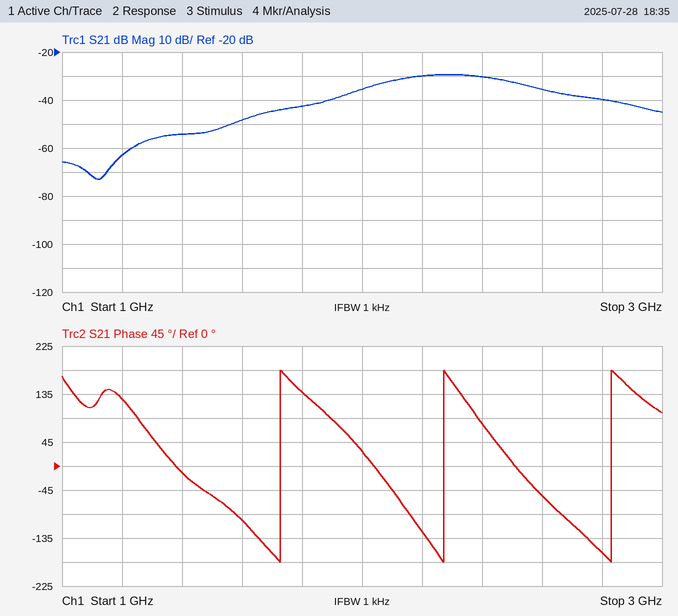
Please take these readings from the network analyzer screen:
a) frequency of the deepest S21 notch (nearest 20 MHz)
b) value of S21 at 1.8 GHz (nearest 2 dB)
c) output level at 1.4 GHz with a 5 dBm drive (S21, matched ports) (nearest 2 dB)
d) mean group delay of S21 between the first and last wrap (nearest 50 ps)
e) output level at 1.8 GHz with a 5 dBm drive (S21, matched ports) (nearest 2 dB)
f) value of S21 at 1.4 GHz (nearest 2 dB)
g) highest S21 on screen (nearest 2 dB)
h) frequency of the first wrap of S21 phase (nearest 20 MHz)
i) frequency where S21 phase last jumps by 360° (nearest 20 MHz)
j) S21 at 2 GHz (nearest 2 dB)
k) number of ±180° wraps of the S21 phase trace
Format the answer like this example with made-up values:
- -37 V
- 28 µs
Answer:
- 1.12 GHz
- -42 dB
- -50 dBm
- 1.80 ns
- -38 dBm
- -54 dB
- -30 dB
- 1.72 GHz
- 2.84 GHz
- -36 dB
- 3
